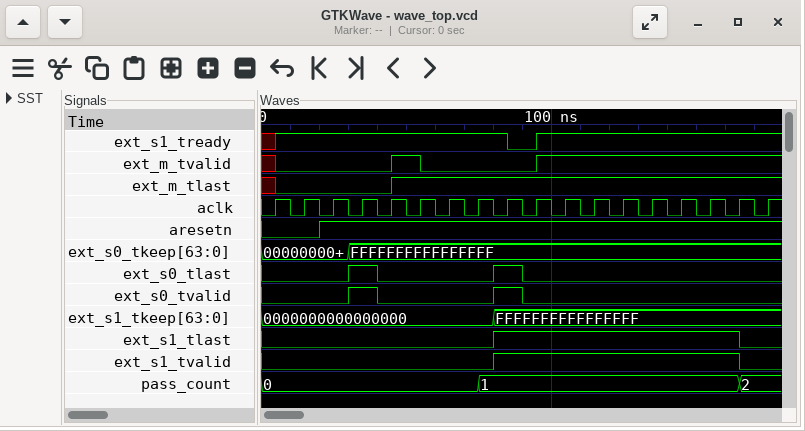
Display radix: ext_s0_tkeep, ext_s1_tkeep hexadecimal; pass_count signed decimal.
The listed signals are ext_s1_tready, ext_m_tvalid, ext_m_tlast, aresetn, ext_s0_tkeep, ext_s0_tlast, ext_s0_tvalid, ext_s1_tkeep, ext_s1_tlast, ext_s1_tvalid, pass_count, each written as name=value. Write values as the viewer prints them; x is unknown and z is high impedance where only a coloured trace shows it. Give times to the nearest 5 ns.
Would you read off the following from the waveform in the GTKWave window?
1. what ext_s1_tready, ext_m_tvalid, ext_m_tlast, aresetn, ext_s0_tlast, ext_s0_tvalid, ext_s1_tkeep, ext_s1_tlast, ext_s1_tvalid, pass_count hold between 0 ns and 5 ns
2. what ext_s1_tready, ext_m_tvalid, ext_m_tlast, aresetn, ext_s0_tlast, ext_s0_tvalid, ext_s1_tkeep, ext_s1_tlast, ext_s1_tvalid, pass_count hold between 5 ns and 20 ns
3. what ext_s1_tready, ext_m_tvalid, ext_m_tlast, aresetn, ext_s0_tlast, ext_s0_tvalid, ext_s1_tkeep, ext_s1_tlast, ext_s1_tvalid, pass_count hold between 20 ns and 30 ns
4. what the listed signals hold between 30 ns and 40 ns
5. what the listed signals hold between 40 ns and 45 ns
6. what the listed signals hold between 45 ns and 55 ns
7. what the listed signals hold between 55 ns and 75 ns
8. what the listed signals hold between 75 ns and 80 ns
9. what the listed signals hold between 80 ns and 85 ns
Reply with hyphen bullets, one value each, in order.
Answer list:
- ext_s1_tready=x, ext_m_tvalid=x, ext_m_tlast=x, aresetn=0, ext_s0_tlast=0, ext_s0_tvalid=0, ext_s1_tkeep=0000000000000000, ext_s1_tlast=0, ext_s1_tvalid=0, pass_count=0
- ext_s1_tready=1, ext_m_tvalid=0, ext_m_tlast=0, aresetn=0, ext_s0_tlast=0, ext_s0_tvalid=0, ext_s1_tkeep=0000000000000000, ext_s1_tlast=0, ext_s1_tvalid=0, pass_count=0
- ext_s1_tready=1, ext_m_tvalid=0, ext_m_tlast=0, aresetn=1, ext_s0_tlast=0, ext_s0_tvalid=0, ext_s1_tkeep=0000000000000000, ext_s1_tlast=0, ext_s1_tvalid=0, pass_count=0
- ext_s1_tready=1, ext_m_tvalid=0, ext_m_tlast=0, aresetn=1, ext_s0_tkeep=FFFFFFFFFFFFFFFF, ext_s0_tlast=1, ext_s0_tvalid=1, ext_s1_tkeep=0000000000000000, ext_s1_tlast=0, ext_s1_tvalid=0, pass_count=0
- ext_s1_tready=1, ext_m_tvalid=0, ext_m_tlast=0, aresetn=1, ext_s0_tkeep=FFFFFFFFFFFFFFFF, ext_s0_tlast=0, ext_s0_tvalid=0, ext_s1_tkeep=0000000000000000, ext_s1_tlast=0, ext_s1_tvalid=0, pass_count=0
- ext_s1_tready=1, ext_m_tvalid=1, ext_m_tlast=1, aresetn=1, ext_s0_tkeep=FFFFFFFFFFFFFFFF, ext_s0_tlast=0, ext_s0_tvalid=0, ext_s1_tkeep=0000000000000000, ext_s1_tlast=0, ext_s1_tvalid=0, pass_count=0
- ext_s1_tready=1, ext_m_tvalid=0, ext_m_tlast=1, aresetn=1, ext_s0_tkeep=FFFFFFFFFFFFFFFF, ext_s0_tlast=0, ext_s0_tvalid=0, ext_s1_tkeep=0000000000000000, ext_s1_tlast=0, ext_s1_tvalid=0, pass_count=0
- ext_s1_tready=1, ext_m_tvalid=0, ext_m_tlast=1, aresetn=1, ext_s0_tkeep=FFFFFFFFFFFFFFFF, ext_s0_tlast=0, ext_s0_tvalid=0, ext_s1_tkeep=0000000000000000, ext_s1_tlast=0, ext_s1_tvalid=0, pass_count=1
- ext_s1_tready=1, ext_m_tvalid=0, ext_m_tlast=1, aresetn=1, ext_s0_tkeep=FFFFFFFFFFFFFFFF, ext_s0_tlast=1, ext_s0_tvalid=1, ext_s1_tkeep=FFFFFFFFFFFFFFFF, ext_s1_tlast=1, ext_s1_tvalid=1, pass_count=1
